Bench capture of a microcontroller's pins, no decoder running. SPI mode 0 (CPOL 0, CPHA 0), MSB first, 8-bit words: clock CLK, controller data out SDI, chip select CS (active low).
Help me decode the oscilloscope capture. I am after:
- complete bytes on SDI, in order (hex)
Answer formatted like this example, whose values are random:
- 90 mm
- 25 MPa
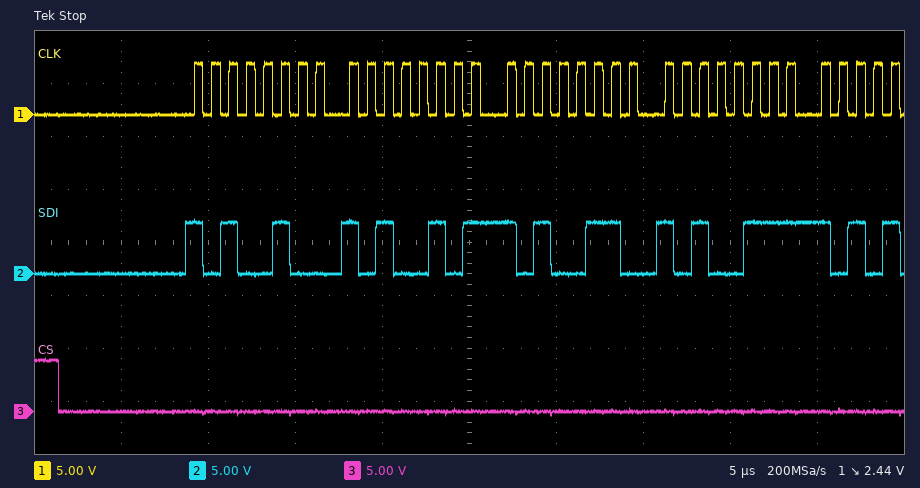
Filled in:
- A4 A5 A6 A7
